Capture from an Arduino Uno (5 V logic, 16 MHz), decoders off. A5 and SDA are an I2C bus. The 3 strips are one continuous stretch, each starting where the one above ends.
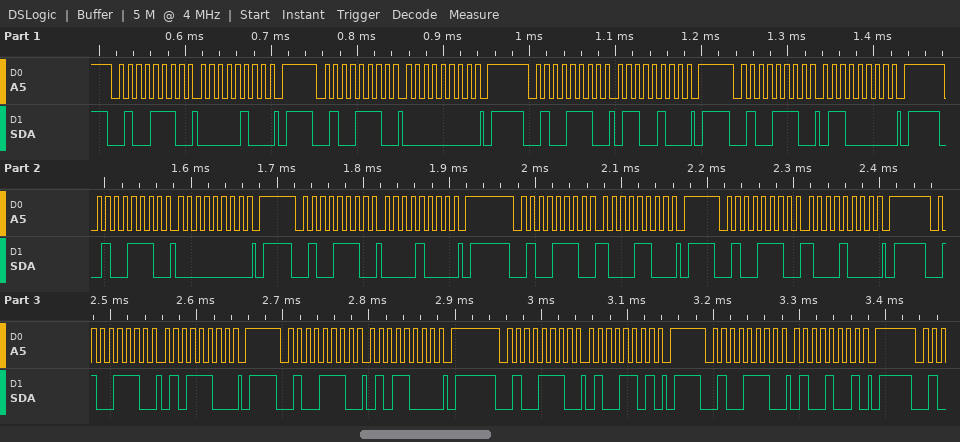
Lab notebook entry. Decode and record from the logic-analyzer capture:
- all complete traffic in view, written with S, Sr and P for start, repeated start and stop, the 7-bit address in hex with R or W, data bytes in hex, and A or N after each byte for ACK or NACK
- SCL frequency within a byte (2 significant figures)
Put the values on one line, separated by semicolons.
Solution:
S 27W A 04 A P S 27W A 00 A P S 27W A 64 A P S 27W A 60 A P S 27W A 00 A P S 27W A 08 A P S 27W A 8C A P S 27W A 88 A P S 27W A 5C A P S 27W A 58 A P S 27W A 4D A P S 27W A 49 A P; 100 kHz
